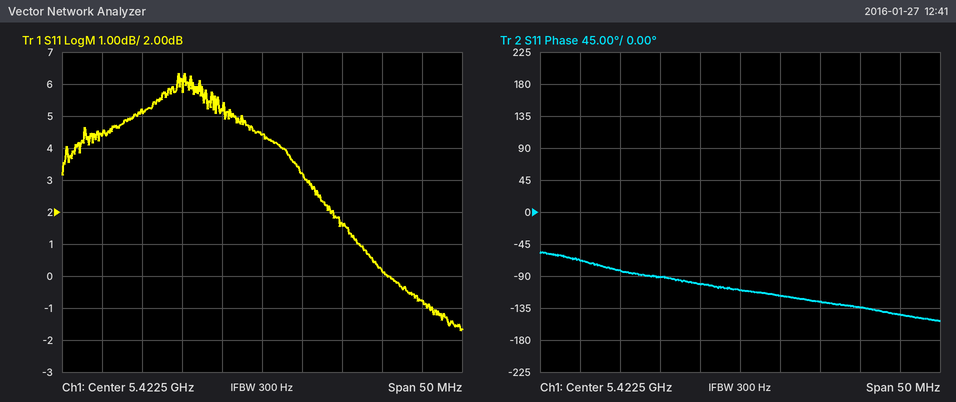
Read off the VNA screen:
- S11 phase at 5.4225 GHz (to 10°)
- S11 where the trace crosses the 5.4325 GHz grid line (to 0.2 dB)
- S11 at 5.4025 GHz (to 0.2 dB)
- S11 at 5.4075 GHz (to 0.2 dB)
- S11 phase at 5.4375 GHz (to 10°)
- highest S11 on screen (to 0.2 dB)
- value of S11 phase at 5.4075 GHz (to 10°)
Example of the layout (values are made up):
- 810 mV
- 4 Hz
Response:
- -110°
- 1.6 dB
- 4.4 dB
- 5.2 dB
- -130°
- 6.4 dB
- -80°
